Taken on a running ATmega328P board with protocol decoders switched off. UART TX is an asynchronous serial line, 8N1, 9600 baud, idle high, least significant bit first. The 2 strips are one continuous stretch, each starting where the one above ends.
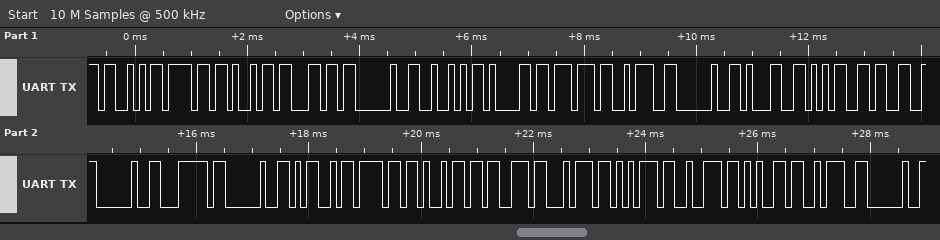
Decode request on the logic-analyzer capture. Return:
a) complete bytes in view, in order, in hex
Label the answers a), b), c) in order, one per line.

a) 53 6F 69 6C 20 52 61 77 3A 20 31 35 33 20 7C 20 4D 6F 69 73 74 75 72 65 3A 20
